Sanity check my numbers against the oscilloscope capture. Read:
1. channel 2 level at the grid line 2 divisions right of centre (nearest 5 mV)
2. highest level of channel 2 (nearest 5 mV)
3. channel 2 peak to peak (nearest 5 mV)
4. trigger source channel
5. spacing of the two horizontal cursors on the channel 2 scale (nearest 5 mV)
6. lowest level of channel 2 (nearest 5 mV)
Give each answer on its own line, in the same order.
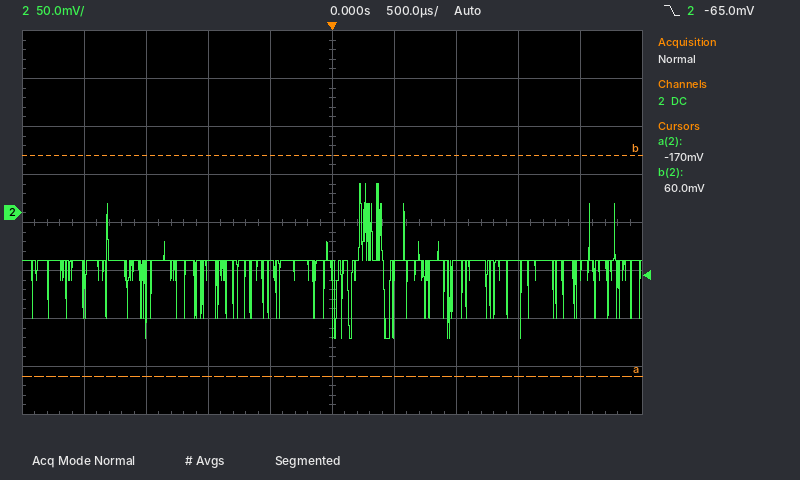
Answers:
-50 mV
30 mV
160 mV
channel 2
230 mV
-130 mV
